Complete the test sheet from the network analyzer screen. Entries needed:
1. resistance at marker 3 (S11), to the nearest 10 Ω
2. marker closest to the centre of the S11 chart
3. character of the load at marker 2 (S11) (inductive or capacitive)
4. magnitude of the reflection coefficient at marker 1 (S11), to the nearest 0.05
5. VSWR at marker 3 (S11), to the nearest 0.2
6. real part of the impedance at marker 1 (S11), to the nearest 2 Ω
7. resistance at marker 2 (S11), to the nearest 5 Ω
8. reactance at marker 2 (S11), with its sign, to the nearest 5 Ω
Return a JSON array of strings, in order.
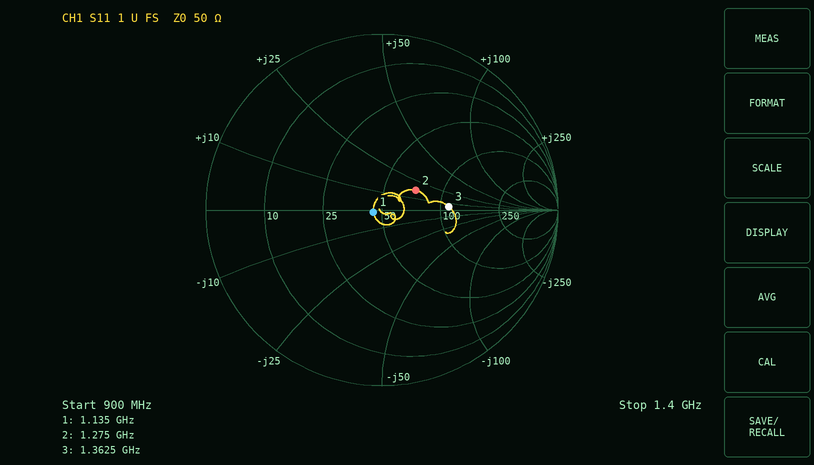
["110 Ω", "marker 1", "inductive", "0.05", "2.2", "46 Ω", "70 Ω", "+15 Ω"]
